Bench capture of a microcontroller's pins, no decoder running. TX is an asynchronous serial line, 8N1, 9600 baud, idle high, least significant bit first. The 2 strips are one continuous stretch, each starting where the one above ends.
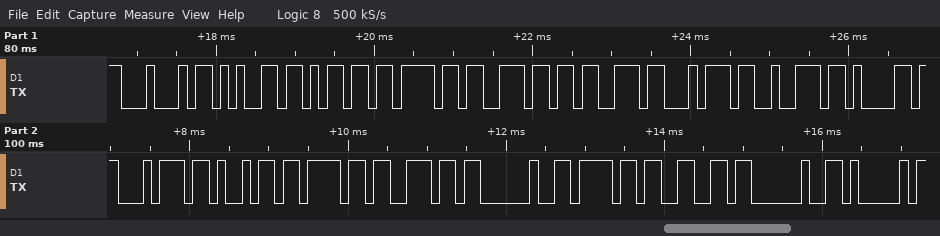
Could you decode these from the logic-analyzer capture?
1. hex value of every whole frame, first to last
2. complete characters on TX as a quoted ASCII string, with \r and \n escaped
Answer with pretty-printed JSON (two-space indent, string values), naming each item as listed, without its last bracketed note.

{
  "hex value of every whole frame, first to last": "44 65 6D 6F 6E 73 74 72 61 74 69 6F 6E 20 6F 66 20 41",
  "complete characters on TX as a quoted ASCII string, with \\r and \\n escaped": "\"Demonstration of A\""
}
